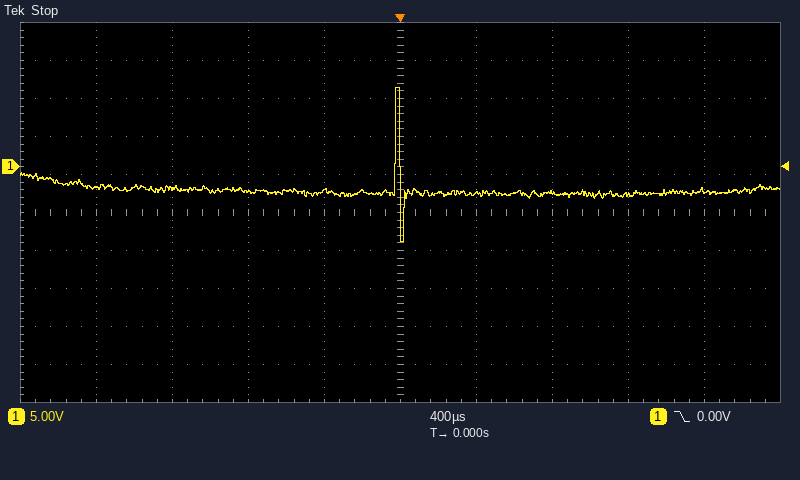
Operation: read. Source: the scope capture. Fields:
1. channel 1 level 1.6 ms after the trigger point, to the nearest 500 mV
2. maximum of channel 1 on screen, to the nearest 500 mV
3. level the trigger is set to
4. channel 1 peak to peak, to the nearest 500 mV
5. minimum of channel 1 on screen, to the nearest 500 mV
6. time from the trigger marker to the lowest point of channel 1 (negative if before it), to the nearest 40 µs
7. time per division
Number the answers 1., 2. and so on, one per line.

1. -3.0 V
2. 10.5 V
3. 0.00 V
4. 20.5 V
5. -10.0 V
6. 0 µs
7. 400 µs
